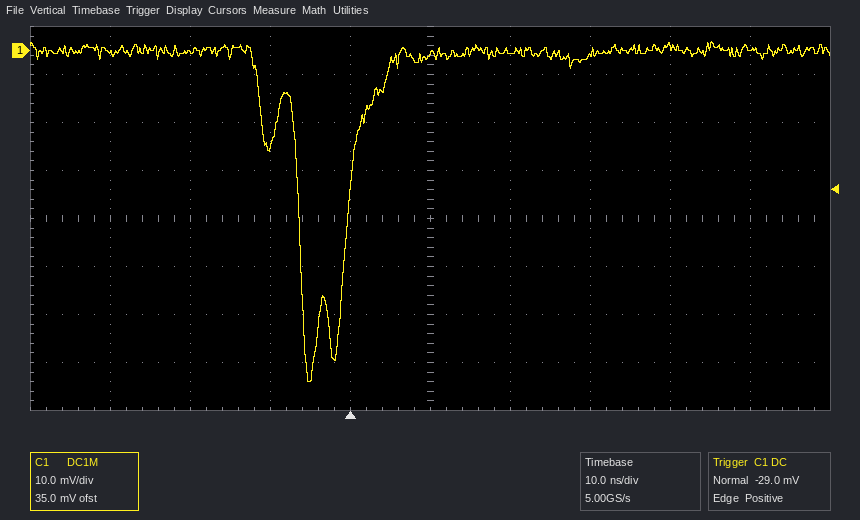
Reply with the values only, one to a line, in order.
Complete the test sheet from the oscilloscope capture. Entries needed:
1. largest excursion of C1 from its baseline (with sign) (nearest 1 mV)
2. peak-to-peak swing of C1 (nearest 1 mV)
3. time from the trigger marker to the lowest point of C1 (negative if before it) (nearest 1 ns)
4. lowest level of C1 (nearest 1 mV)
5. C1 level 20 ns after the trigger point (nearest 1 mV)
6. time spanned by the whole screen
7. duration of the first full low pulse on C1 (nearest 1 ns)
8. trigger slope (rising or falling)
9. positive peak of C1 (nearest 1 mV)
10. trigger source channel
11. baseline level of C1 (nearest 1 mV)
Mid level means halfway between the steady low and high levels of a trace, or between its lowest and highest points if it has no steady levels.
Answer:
-69 mV
71 mV
-5 ns
-69 mV
0 mV
100 ns
6 ns
rising
2 mV
C1
0 mV
